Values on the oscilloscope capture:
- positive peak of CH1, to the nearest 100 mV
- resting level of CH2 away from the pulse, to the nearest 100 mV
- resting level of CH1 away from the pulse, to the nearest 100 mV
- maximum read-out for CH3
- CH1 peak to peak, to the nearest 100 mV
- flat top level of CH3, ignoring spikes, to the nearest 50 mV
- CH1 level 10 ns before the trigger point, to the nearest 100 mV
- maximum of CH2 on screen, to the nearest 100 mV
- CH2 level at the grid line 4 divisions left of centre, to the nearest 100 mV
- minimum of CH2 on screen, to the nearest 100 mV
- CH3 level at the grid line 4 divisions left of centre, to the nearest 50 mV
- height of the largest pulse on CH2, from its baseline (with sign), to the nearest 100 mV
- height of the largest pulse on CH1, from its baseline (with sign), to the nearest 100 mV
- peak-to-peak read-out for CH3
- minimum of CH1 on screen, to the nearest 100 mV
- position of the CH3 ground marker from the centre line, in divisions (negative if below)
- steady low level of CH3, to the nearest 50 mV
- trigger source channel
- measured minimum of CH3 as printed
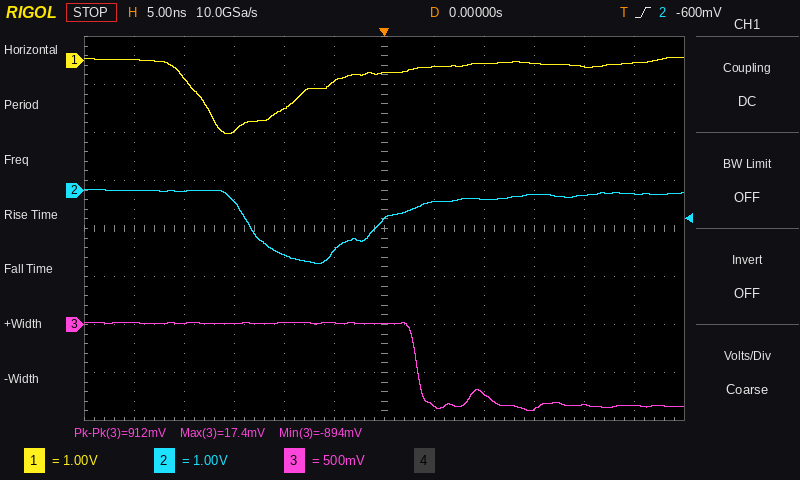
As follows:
100 mV
-100 mV
-100 mV
17.4 mV
1.6 V
0 mV
-1.0 V
0.0 V
0.0 V
-1.5 V
0 mV
-1.4 V
-1.4 V
912 mV
-1.5 V
-2.0 div
-850 mV
CH2
-894 mV
